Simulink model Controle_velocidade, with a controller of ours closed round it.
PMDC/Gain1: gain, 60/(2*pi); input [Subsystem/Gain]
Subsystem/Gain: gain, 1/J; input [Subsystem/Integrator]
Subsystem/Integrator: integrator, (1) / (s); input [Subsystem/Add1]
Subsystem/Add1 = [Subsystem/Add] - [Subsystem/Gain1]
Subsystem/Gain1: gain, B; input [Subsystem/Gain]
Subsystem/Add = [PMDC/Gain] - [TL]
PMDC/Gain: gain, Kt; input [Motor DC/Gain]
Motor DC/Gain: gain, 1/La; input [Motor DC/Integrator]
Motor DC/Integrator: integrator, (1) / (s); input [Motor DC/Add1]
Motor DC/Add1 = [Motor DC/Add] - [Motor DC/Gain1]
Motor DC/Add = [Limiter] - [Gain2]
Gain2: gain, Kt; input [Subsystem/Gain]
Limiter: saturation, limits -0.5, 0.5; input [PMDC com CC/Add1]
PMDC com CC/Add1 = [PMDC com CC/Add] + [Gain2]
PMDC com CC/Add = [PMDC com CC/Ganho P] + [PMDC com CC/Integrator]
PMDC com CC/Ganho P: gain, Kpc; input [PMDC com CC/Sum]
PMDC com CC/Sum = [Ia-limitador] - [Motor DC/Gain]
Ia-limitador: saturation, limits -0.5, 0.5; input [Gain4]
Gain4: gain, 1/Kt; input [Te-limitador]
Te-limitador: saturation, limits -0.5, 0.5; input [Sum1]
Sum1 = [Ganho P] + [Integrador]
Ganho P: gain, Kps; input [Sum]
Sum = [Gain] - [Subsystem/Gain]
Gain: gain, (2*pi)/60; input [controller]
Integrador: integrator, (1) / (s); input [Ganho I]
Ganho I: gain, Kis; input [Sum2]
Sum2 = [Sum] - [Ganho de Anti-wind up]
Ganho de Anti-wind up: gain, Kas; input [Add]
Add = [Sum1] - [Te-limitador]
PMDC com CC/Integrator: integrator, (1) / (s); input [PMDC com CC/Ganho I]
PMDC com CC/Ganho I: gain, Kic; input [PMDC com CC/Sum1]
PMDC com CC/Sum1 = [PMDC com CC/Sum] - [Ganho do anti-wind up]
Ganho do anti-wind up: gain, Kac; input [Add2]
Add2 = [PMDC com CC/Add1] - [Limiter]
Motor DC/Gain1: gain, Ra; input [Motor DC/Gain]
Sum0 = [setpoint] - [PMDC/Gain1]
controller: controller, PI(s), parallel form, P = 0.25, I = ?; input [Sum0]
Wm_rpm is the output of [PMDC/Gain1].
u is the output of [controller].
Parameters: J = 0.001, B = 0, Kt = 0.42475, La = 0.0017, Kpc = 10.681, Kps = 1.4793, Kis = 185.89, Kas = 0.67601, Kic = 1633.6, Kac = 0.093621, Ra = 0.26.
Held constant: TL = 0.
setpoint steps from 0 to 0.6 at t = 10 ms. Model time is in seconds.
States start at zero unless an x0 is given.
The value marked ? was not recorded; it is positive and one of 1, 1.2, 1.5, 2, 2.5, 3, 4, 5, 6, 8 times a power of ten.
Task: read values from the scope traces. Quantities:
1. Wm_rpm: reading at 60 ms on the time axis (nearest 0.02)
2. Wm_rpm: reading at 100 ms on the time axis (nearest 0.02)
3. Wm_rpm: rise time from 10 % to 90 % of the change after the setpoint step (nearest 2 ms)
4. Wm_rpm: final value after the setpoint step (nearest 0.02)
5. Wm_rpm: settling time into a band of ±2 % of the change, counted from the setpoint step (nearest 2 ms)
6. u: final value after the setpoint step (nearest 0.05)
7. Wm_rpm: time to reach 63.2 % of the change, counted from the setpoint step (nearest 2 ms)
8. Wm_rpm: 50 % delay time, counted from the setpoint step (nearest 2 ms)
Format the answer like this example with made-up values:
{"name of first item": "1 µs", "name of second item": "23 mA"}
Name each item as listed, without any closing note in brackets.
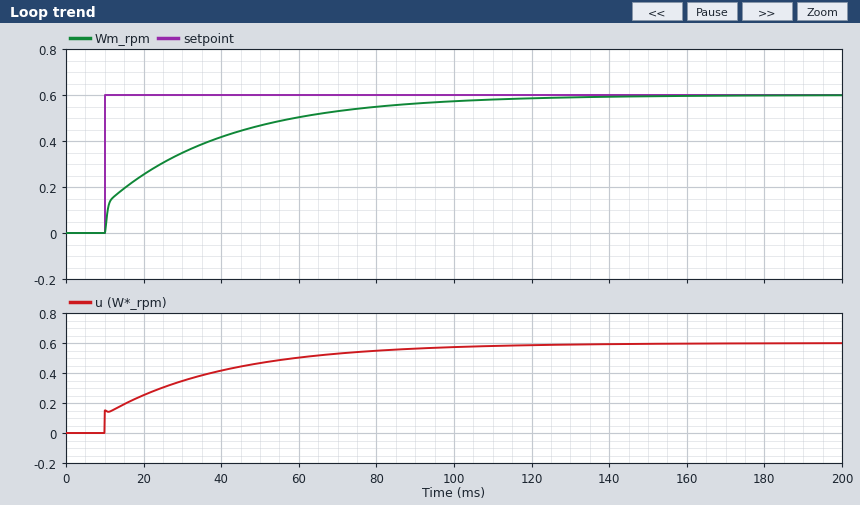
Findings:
{"Wm_rpm: reading at 60 ms on the time axis": "0.50", "Wm_rpm: reading at 100 ms on the time axis": "0.58", "Wm_rpm: rise time from 10 % to 90 % of the change after the setpoint step": "64 ms", "Wm_rpm: final value after the setpoint step": "0.60", "Wm_rpm: settling time into a band of ±2 % of the change, counted from the setpoint step": "116 ms", "u: final value after the setpoint step": "0.60", "Wm_rpm: time to reach 63.2 % of the change, counted from the setpoint step": "24 ms", "Wm_rpm: 50 % delay time, counted from the setpoint step": "14 ms"}
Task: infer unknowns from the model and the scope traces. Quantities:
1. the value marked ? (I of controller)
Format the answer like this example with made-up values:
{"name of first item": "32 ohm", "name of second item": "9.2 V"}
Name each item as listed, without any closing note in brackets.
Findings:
{"the value marked ?": "40"}
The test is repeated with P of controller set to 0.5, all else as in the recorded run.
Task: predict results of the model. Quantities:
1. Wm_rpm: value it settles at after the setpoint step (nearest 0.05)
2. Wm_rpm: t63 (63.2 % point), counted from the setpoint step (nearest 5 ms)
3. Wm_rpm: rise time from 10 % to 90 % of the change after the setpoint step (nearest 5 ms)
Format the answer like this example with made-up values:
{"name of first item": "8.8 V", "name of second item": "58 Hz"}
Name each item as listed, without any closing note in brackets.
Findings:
{"Wm_rpm: value it settles at after the setpoint step": "0.60", "Wm_rpm: t63 (63.2 % point), counted from the setpoint step": "20 ms", "Wm_rpm: rise time from 10 % to 90 % of the change after the setpoint step": "70 ms"}
